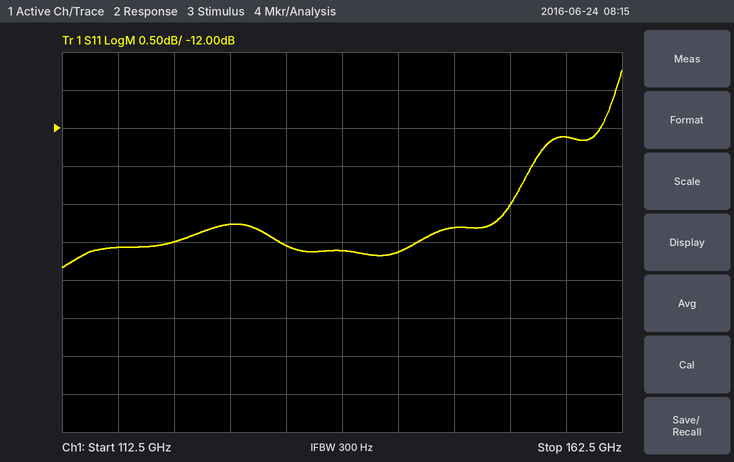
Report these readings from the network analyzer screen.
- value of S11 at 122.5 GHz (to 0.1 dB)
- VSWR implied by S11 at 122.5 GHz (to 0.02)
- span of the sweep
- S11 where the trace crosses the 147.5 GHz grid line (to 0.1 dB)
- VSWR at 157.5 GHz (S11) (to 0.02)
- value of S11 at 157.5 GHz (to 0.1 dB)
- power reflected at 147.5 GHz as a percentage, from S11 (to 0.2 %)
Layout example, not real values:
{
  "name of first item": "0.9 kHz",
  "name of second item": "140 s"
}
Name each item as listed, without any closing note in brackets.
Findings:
{
  "value of S11 at 122.5 GHz": "-13.5 dB",
  "VSWR implied by S11 at 122.5 GHz": "1.54",
  "span of the sweep": "50 GHz",
  "S11 where the trace crosses the 147.5 GHz grid line": "-13.3 dB",
  "VSWR at 157.5 GHz (S11)": "1.66",
  "value of S11 at 157.5 GHz": "-12.1 dB",
  "power reflected at 147.5 GHz as a percentage, from S11": "4.6 %"
}
